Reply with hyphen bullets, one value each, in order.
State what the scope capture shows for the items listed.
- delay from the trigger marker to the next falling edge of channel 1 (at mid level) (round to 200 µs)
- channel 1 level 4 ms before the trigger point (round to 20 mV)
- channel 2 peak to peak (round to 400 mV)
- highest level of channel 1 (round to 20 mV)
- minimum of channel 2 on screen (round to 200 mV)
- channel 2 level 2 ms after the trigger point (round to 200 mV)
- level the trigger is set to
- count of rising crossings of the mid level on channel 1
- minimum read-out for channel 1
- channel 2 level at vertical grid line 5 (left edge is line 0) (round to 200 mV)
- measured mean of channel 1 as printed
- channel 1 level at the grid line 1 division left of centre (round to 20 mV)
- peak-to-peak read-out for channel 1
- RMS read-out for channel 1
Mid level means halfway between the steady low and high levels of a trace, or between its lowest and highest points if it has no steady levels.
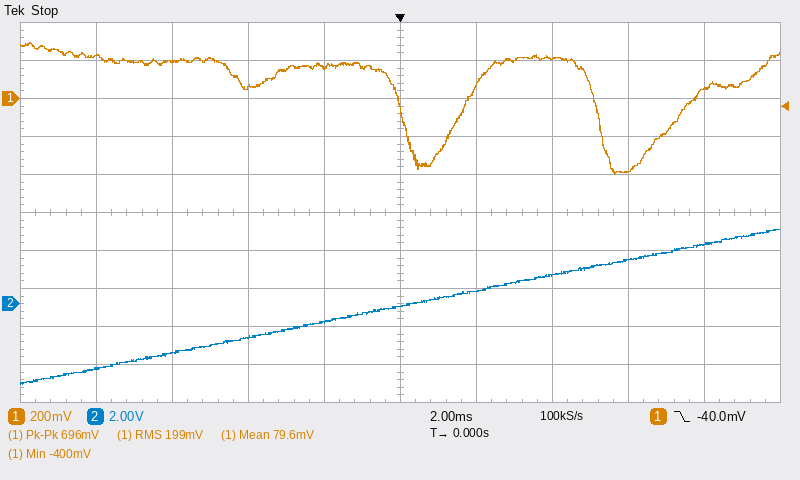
- 5.2 ms
- 60 mV
- 8.0 V
- 300 mV
- -4.2 V
- 600 mV
- -40.0 mV
- 2
- -400 mV
- -200 mV
- 79.6 mV
- 160 mV
- 696 mV
- 199 mV
